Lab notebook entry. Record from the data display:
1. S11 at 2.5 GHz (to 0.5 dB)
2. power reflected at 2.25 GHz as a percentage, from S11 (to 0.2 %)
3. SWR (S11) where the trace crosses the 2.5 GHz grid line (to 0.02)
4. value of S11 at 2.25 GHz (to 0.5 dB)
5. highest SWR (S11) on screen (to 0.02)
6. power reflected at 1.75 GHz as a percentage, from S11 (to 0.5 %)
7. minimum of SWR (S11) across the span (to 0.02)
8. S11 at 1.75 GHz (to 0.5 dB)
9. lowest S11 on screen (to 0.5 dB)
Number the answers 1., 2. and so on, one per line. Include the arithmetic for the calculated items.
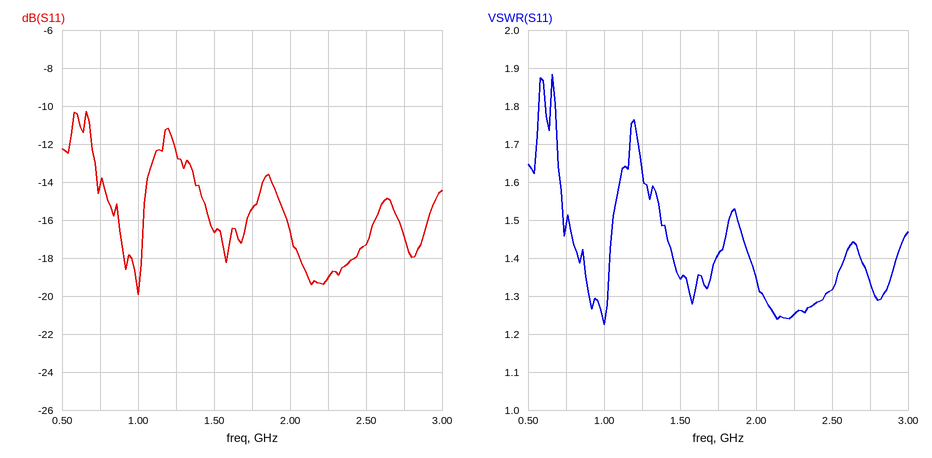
1. -17.5 dB
2. 10^(-19/10) ≈ 1.26 %, so 1.2 % to the nearest 0.2 %
3. 1.32
4. -19.0 dB
5. 1.88
6. 10^(-15.5/10) ≈ 2.82 %, so 3.0 % to the nearest 0.5 %
7. 1.22
8. -15.5 dB
9. -20.0 dB
